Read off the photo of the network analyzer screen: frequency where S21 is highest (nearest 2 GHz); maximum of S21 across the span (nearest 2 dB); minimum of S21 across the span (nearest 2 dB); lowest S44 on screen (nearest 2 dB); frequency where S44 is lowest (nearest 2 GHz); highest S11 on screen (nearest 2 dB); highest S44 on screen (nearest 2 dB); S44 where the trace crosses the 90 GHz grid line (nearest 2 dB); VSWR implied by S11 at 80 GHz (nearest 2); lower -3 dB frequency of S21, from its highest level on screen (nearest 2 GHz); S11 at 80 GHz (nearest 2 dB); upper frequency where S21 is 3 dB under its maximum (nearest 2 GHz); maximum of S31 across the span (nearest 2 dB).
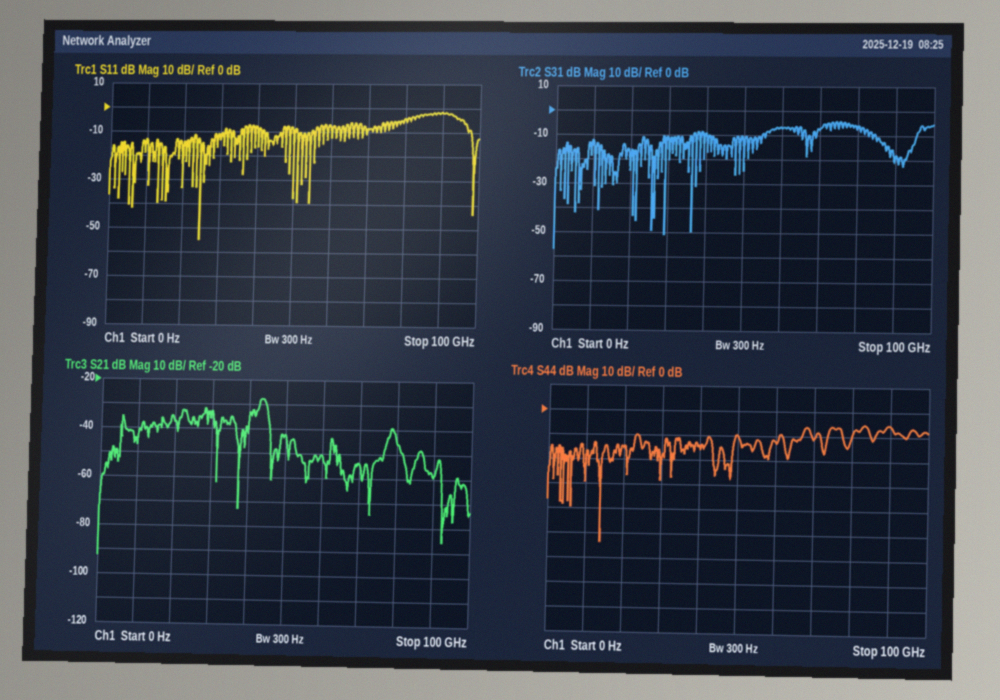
44 GHz
-28 dB
-92 dB
-54 dB
14 GHz
-2 dB
-6 dB
-6 dB
4
42 GHz
-4 dB
44 GHz
-4 dB
